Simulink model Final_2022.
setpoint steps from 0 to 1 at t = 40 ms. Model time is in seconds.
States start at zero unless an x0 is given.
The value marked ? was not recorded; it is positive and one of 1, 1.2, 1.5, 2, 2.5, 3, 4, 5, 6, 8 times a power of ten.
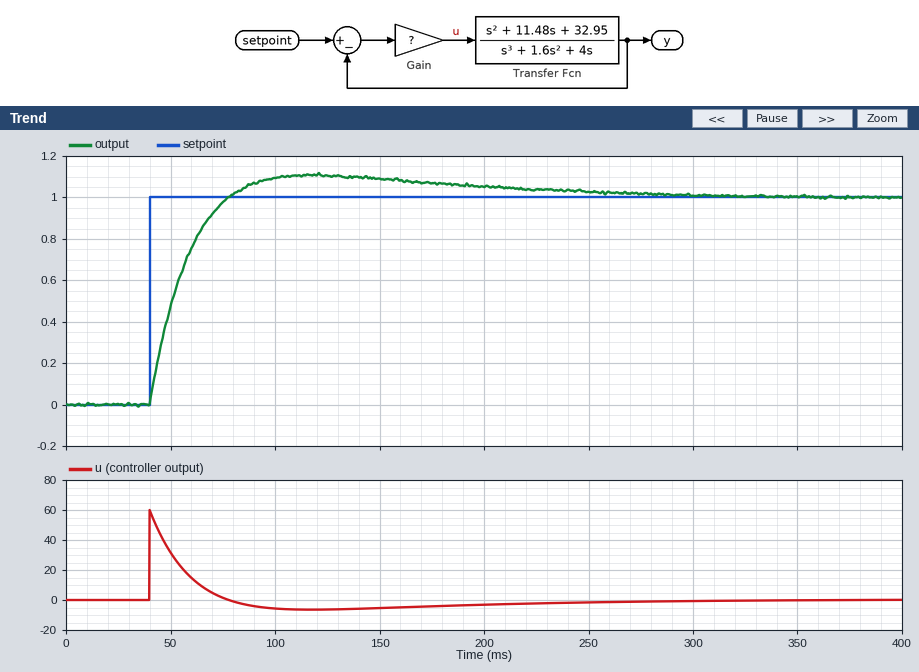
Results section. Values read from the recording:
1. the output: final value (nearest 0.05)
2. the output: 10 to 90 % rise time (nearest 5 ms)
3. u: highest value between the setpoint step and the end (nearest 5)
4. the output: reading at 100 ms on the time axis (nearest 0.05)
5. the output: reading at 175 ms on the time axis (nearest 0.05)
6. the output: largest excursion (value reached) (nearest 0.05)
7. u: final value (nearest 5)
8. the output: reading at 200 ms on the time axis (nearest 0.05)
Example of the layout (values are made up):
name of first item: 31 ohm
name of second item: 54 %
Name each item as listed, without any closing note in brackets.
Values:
the output: final value: 1.00
the output: 10 to 90 % rise time: 25 ms
u: highest value between the setpoint step and the end: 60
the output: reading at 100 ms on the time axis: 1.10
the output: reading at 175 ms on the time axis: 1.05
the output: largest excursion (value reached): 1.10
u: final value: 0
the output: reading at 200 ms on the time axis: 1.05
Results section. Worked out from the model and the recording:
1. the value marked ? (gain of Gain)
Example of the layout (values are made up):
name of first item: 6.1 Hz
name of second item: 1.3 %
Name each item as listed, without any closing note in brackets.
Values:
the value marked ?: 60
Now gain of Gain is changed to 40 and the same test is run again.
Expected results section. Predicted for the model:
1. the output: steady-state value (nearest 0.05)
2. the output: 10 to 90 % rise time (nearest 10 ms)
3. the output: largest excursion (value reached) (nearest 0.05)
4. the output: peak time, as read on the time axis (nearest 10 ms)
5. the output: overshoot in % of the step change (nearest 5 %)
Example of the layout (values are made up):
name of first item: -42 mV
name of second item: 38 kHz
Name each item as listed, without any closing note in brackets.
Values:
the output: steady-state value: 1.00
the output: 10 to 90 % rise time: 40 ms
the output: largest excursion (value reached): 1.15
the output: peak time, as read on the time axis: 140 ms
the output: overshoot in % of the step change: 15 %
